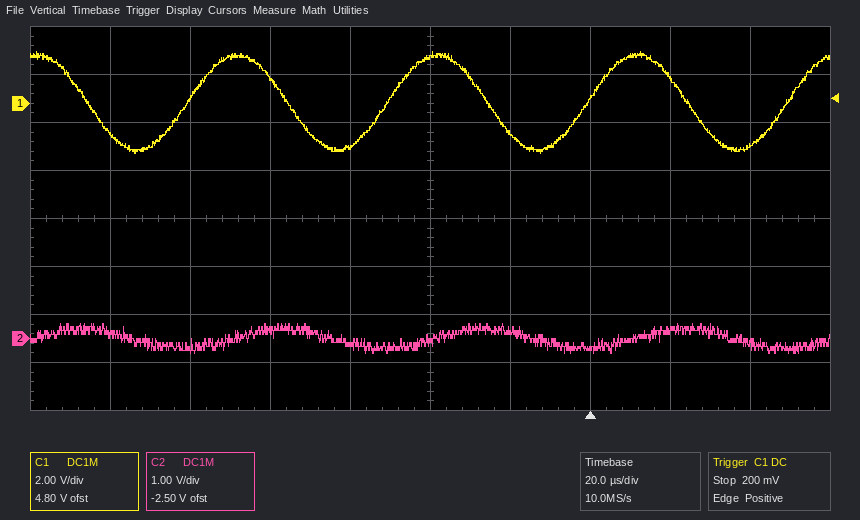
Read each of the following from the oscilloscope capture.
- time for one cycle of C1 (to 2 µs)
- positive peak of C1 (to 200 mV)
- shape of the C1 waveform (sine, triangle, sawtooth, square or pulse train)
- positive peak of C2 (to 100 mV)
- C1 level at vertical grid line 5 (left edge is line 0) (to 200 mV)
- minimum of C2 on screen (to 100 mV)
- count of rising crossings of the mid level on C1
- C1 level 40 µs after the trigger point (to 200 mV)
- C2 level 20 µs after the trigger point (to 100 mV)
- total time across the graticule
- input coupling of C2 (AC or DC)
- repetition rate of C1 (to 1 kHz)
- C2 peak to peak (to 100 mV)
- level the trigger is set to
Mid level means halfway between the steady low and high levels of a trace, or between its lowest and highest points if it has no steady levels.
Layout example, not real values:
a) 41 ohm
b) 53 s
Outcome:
a) 50 µs
b) 2.2 V
c) sine
d) 300 mV
e) 2.0 V
f) -300 mV
g) 4
h) -1.8 V
i) 200 mV
j) 200 µs
k) DC
l) 20 kHz
m) 600 mV
n) 200 mV
